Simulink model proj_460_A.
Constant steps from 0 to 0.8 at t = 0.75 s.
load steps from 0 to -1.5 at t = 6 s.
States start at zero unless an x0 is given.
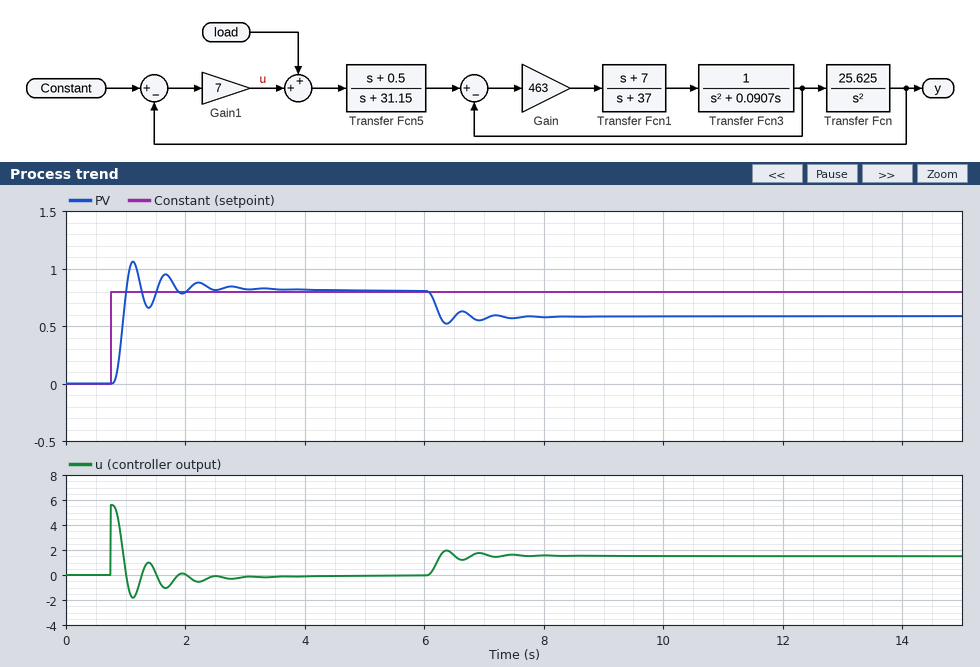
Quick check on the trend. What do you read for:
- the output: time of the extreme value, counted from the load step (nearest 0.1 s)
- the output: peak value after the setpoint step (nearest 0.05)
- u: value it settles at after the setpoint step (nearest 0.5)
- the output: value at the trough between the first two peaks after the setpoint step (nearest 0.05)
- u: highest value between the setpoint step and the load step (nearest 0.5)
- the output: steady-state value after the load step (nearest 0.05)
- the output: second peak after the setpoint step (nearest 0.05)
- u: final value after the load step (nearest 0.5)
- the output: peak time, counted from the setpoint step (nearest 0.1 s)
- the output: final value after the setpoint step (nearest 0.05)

0.4 s
1.05
0.0
0.65
5.5
0.60
0.95
1.5
0.4 s
0.80
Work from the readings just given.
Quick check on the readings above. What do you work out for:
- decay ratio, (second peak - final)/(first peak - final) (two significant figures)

0.60
